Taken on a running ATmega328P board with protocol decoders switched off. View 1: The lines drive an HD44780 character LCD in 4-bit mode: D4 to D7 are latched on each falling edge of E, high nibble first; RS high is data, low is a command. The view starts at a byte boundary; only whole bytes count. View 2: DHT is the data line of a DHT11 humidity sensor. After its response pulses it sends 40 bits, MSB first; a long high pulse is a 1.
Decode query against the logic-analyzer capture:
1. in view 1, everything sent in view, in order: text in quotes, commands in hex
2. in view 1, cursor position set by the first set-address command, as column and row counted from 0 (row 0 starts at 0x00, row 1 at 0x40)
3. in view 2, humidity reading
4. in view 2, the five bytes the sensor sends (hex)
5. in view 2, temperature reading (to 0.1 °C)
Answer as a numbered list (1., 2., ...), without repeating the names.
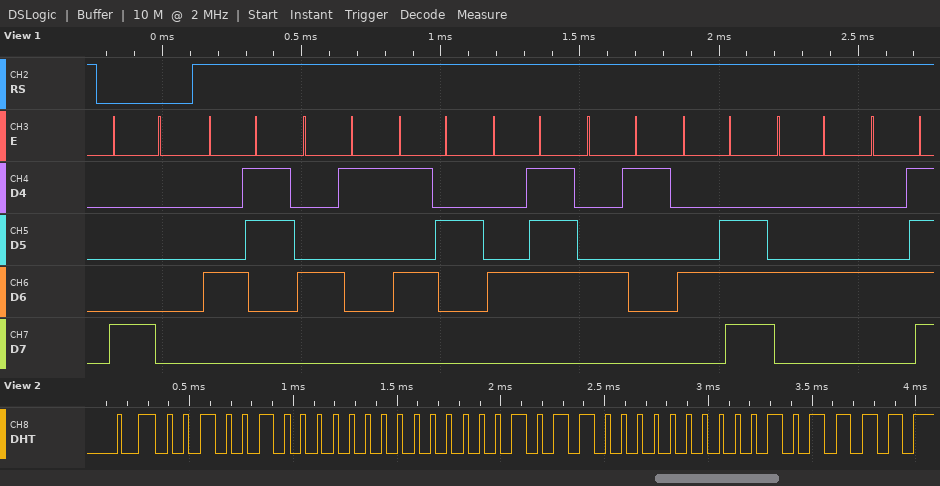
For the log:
1. 0x80 "CARGANDO"
2. column 0, row 0
3. 36 %
4. 24 00 0B 00 2F
5. 11.0 °C
